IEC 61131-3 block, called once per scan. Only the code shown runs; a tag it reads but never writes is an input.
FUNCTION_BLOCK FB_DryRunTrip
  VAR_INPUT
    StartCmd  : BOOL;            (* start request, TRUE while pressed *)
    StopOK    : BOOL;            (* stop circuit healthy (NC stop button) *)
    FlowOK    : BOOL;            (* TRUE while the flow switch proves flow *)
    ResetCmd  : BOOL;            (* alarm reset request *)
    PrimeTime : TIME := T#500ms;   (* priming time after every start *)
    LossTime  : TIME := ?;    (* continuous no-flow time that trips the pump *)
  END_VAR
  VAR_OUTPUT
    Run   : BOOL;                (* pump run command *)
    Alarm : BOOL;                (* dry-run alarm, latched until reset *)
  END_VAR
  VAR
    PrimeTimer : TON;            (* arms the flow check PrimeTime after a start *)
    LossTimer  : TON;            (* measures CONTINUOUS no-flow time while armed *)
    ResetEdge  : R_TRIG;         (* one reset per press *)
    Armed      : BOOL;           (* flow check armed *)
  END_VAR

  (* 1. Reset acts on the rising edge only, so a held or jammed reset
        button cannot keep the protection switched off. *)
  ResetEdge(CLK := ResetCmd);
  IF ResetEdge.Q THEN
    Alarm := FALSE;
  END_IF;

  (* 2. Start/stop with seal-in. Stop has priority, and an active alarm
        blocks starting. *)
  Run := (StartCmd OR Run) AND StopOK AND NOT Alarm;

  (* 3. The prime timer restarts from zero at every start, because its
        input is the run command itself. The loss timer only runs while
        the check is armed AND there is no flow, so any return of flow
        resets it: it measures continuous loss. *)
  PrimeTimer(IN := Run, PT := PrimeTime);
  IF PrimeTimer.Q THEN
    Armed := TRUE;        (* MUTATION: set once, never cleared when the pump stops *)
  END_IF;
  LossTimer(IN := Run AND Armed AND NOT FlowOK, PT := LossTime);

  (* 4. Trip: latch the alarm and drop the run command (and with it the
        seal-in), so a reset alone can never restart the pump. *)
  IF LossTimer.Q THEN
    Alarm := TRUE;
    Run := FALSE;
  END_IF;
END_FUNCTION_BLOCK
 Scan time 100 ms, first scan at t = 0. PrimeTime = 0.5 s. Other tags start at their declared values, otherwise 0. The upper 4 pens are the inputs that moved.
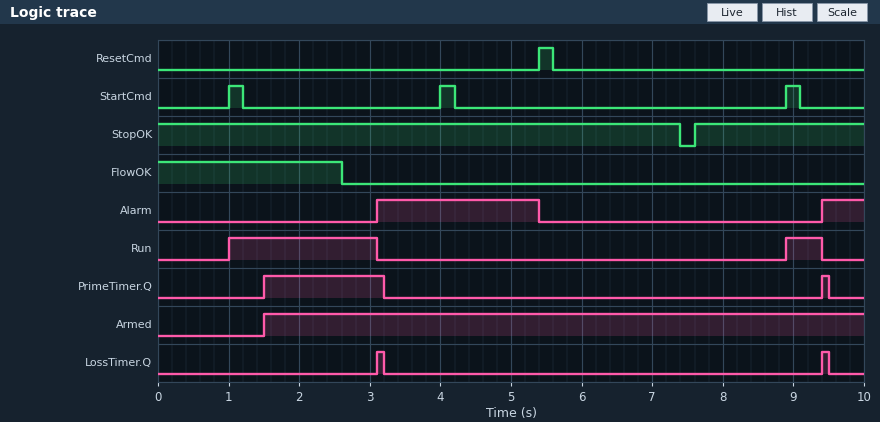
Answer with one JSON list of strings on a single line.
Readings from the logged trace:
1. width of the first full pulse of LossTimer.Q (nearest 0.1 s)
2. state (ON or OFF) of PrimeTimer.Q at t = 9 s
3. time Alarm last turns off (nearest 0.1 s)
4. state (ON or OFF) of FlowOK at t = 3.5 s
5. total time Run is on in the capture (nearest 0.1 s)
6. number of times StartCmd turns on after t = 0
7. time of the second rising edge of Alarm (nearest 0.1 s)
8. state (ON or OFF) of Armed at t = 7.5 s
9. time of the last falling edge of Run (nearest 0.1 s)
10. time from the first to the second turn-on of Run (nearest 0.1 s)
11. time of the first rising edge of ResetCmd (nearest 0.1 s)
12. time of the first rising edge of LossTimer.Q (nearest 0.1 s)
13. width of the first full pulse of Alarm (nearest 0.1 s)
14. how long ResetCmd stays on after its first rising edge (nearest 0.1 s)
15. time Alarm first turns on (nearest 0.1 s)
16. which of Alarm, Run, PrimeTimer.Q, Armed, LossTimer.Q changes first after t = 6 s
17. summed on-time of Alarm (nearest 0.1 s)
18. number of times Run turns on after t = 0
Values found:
["0.1 s", "OFF", "5.4 s", "OFF", "2.6 s", "3", "9.4 s", "ON", "9.4 s", "7.9 s", "5.4 s", "3.1 s", "2.3 s", "0.2 s", "3.1 s", "Run", "2.9 s", "2"]
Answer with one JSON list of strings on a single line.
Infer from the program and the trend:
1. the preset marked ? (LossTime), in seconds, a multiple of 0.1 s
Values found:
["0.5 s"]
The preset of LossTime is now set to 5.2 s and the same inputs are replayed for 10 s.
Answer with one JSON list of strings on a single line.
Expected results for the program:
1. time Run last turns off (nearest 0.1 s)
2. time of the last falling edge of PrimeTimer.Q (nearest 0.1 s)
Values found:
["7.4 s", "7.4 s"]
